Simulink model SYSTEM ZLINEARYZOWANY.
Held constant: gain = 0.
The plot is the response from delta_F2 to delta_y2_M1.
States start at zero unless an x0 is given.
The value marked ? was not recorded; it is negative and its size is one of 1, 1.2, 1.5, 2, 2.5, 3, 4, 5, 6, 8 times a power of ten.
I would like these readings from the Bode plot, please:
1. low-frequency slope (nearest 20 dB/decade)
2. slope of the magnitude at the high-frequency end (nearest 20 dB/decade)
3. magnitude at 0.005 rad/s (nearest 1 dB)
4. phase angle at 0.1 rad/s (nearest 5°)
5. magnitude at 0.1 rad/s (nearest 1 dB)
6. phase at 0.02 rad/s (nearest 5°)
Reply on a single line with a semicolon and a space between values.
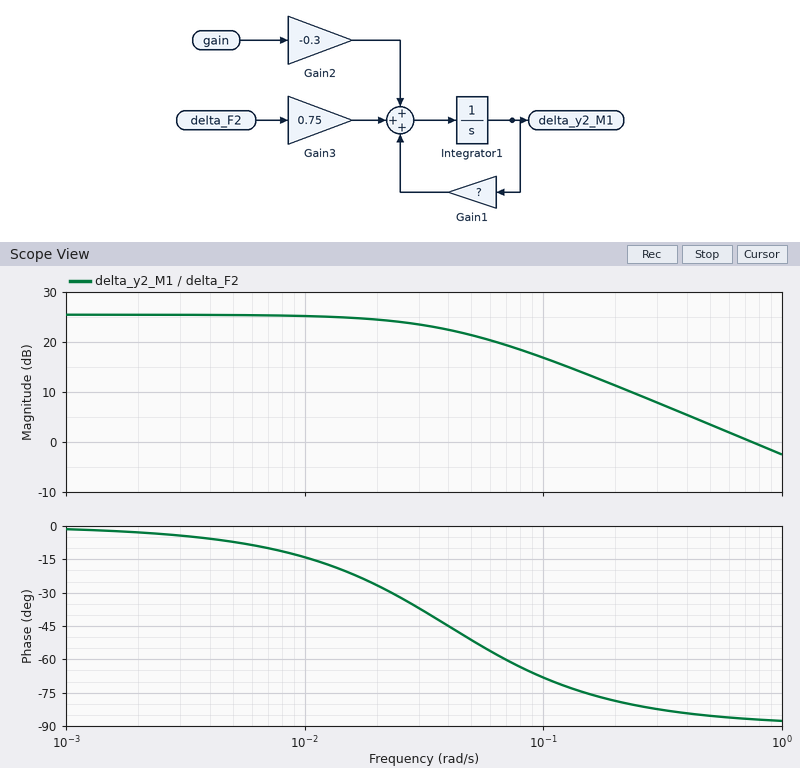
0 dB/decade; -20 dB/decade; 25 dB; -70°; 17 dB; -25°
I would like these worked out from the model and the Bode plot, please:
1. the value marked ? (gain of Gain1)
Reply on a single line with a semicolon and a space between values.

-0.04
